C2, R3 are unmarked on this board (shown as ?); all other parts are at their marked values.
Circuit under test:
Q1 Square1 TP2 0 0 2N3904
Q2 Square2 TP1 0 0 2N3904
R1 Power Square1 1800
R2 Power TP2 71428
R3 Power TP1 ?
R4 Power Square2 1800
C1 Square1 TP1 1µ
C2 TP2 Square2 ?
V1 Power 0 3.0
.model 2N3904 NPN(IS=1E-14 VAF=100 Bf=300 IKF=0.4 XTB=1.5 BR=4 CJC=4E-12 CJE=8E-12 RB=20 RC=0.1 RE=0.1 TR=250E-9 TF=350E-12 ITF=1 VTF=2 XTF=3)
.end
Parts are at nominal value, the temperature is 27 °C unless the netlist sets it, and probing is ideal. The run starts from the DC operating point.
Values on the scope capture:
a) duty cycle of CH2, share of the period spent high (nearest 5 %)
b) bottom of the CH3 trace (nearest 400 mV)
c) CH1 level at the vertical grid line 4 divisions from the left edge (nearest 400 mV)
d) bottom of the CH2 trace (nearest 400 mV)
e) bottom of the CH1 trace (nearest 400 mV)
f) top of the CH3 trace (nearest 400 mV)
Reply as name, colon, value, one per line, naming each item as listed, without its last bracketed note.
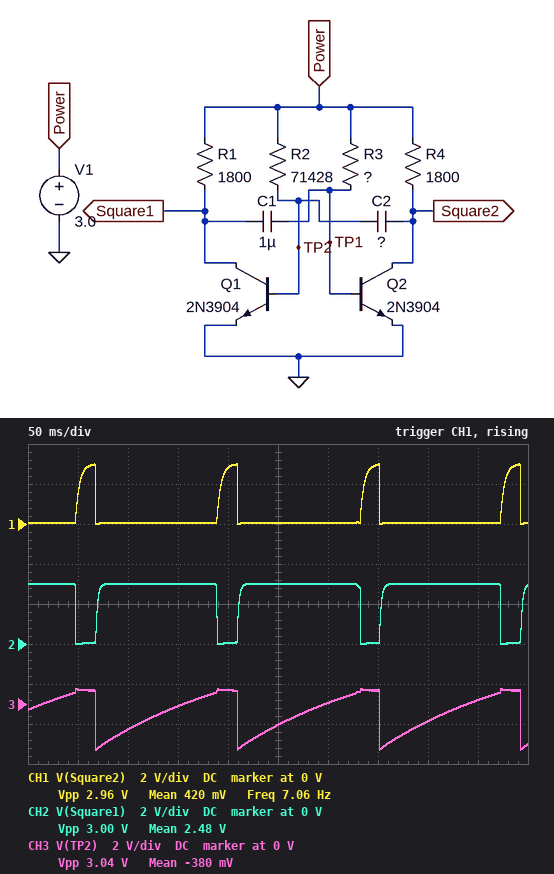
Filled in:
duty cycle of CH2, share of the period spent high: 85 %
bottom of the CH3 trace: -2.4 V
CH1 level at the vertical grid line 4 divisions from the left edge: 2.8 V
bottom of the CH2 trace: 0 V
bottom of the CH1 trace: 0 V
top of the CH3 trace: 800 mV
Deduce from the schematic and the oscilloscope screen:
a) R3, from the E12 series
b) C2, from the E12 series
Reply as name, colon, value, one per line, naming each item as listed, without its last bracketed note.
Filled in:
R3, from the E12 series: 27 kΩ
C2, from the E12 series: 2.2 µF
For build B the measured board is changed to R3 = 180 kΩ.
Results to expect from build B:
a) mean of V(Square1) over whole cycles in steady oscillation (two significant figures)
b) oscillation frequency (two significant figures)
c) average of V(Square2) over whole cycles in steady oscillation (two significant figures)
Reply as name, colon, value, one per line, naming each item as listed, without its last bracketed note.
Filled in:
mean of V(Square1) over whole cycles in steady oscillation: 1.4 V
oscillation frequency: 4.0 Hz
average of V(Square2) over whole cycles in steady oscillation: 1.6 V
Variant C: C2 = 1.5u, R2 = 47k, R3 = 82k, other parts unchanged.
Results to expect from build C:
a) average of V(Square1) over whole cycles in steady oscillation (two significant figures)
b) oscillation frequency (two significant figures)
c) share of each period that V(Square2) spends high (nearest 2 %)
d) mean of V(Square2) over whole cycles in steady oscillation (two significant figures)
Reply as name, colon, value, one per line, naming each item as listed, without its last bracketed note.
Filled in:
average of V(Square1) over whole cycles in steady oscillation: 1.4 V
oscillation frequency: 8.7 Hz
share of each period that V(Square2) spends high: 52 %
mean of V(Square2) over whole cycles in steady oscillation: 1.6 V
